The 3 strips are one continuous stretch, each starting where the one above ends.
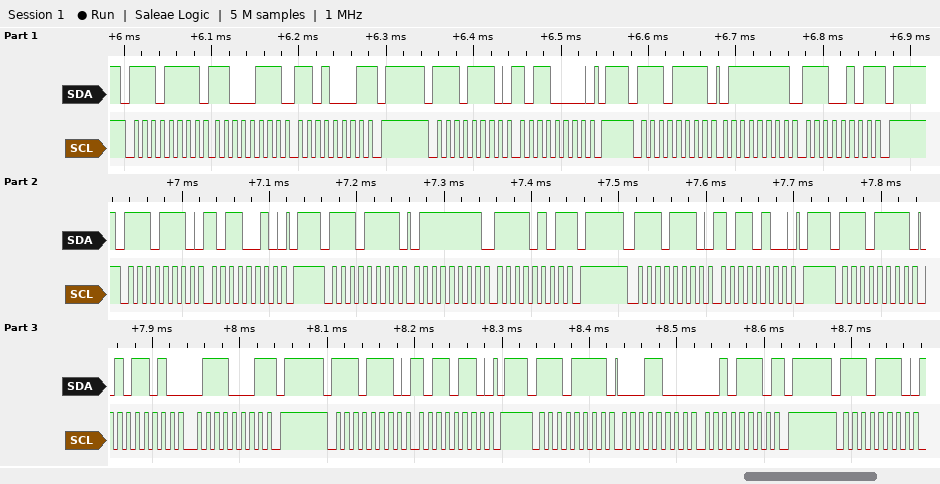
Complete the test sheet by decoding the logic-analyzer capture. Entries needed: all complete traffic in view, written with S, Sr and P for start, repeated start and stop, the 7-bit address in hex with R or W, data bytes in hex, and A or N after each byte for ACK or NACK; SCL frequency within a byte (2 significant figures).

S 77R A C7 A D1 N P S 77W A B0 A P S 77R A 7F A E5 N P S 77W A B2 A P S 77R A 7F A F5 N P S 77W A B4 A P S 77R A 5A A 71 N P S 77W A B6 A P S 77R A 18 A 2E N P S 77W A
100 kHz
